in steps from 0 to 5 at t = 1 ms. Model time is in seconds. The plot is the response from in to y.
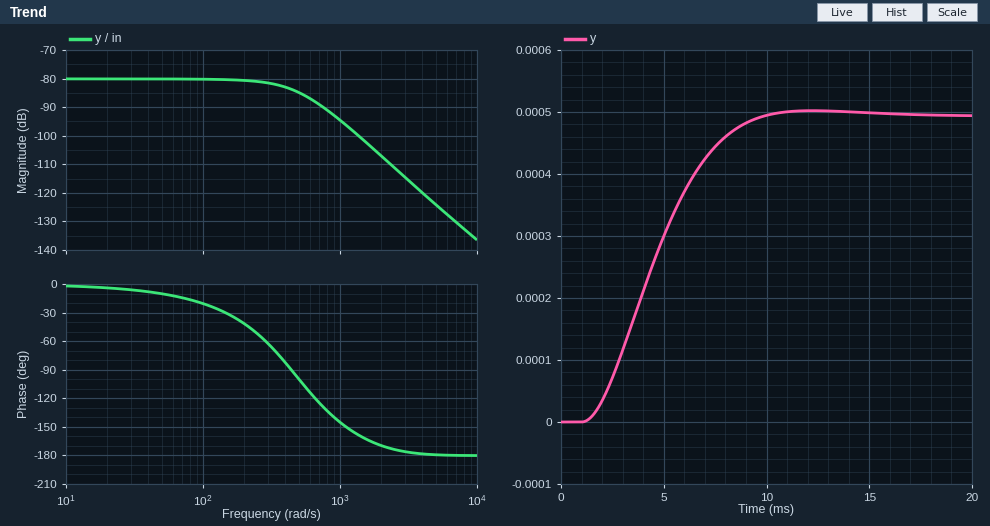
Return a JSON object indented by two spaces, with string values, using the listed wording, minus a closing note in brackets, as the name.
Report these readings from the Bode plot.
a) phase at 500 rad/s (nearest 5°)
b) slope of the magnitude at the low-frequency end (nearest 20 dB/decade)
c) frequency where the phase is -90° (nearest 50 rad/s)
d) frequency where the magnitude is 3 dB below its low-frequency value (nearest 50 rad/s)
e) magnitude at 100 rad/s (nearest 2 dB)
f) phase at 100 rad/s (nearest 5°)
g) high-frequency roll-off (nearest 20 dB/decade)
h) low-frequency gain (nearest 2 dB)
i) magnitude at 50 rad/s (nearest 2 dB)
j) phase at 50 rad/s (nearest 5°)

{
  "phase at 500 rad/s": "-100°",
  "slope of the magnitude at the low-frequency end": "0 dB/decade",
  "frequency where the phase is -90°": "450 rad/s",
  "frequency where the magnitude is 3 dB below its low-frequency value": "400 rad/s",
  "magnitude at 100 rad/s": "-80 dB",
  "phase at 100 rad/s": "-20°",
  "high-frequency roll-off": "-40 dB/decade",
  "low-frequency gain": "-80 dB",
  "magnitude at 50 rad/s": "-80 dB",
  "phase at 50 rad/s": "-10°"
}
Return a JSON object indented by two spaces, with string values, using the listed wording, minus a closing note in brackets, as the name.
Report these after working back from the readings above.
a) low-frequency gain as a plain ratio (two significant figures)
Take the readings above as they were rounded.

{
  "low-frequency gain as a plain ratio": "0.00010"
}
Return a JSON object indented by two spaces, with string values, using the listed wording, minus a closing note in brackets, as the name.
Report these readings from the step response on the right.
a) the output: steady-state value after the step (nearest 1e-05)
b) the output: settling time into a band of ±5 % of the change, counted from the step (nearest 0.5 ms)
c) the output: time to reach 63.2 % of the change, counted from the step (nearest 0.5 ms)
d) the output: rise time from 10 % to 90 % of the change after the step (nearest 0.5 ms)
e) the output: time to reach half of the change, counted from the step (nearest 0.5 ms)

{
  "the output: steady-state value after the step": "0.00049",
  "the output: settling time into a band of ±5 % of the change, counted from the step": "7.5 ms",
  "the output: time to reach 63.2 % of the change, counted from the step": "4.0 ms",
  "the output: rise time from 10 % to 90 % of the change after the step": "5.5 ms",
  "the output: time to reach half of the change, counted from the step": "3.5 ms"
}
